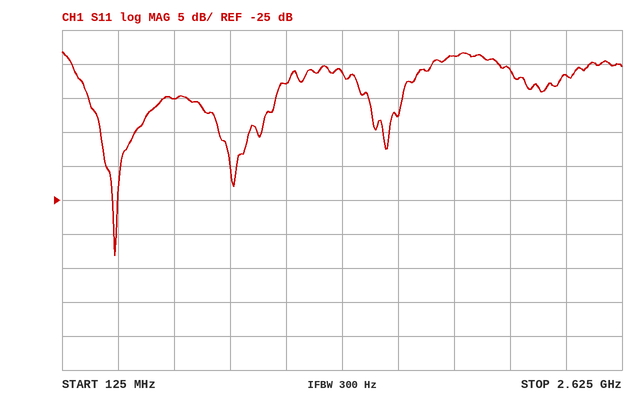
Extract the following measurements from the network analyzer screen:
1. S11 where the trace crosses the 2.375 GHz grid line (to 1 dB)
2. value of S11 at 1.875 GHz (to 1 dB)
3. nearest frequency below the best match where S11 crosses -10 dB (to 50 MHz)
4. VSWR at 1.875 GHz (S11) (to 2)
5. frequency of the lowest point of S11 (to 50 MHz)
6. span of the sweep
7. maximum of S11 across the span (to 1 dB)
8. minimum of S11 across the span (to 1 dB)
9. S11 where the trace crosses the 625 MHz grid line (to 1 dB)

-7 dB
-4 dB
250 MHz
4
350 MHz
2.5 GHz
-3 dB
-33 dB
-10 dB
